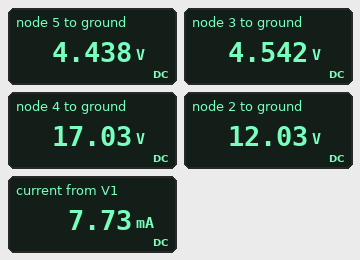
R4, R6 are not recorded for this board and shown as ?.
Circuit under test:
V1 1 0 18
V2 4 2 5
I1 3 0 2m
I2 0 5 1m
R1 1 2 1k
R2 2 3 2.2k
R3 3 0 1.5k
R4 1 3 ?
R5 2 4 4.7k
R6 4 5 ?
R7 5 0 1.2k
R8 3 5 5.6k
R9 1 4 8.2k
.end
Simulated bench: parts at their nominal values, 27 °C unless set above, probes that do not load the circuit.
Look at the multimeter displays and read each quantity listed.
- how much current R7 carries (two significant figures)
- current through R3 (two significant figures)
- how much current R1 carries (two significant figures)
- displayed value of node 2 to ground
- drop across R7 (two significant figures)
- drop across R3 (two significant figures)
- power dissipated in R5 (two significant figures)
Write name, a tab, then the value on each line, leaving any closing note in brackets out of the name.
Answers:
how much current R7 carries	3.7 mA
current through R3	3.0 mA
how much current R1 carries	6.0 mA
displayed value of node 2 to ground	12.03 V
drop across R7	4.4 V
drop across R3	4.5 V
power dissipated in R5	5.3 mW
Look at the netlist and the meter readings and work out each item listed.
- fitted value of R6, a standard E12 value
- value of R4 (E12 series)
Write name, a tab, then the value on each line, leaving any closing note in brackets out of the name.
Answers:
fitted value of R6, a standard E12 value	4.7 kΩ
value of R4	8.2 kΩ
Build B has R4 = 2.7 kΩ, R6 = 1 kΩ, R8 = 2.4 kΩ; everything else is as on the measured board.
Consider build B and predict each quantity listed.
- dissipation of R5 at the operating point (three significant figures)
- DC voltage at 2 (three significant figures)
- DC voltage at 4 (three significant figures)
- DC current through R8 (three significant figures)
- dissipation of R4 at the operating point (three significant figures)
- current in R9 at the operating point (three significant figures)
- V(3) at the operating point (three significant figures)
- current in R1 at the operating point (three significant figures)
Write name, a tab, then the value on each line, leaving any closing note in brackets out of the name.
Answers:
dissipation of R5 at the operating point	5.32 mW
DC voltage at 2	10.1 V
DC voltage at 4	15.1 V
DC current through R8	712 µA
dissipation of R4 at the operating point	47.4 mW
current in R9 at the operating point	354 µA
V(3) at the operating point	6.68 V
current in R1 at the operating point	7.90 mA
